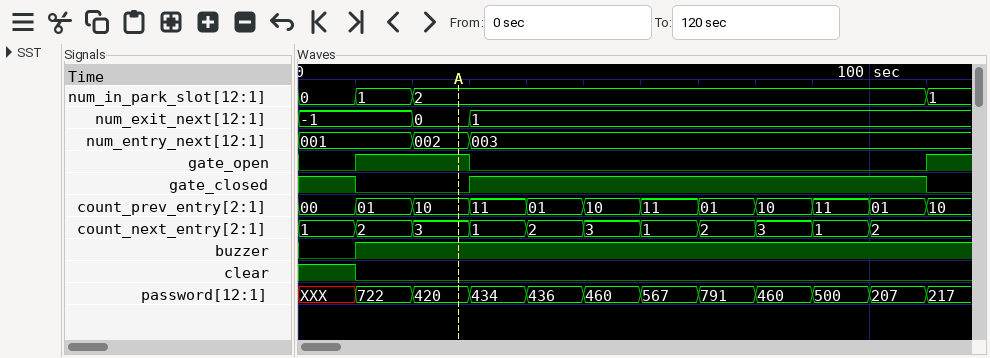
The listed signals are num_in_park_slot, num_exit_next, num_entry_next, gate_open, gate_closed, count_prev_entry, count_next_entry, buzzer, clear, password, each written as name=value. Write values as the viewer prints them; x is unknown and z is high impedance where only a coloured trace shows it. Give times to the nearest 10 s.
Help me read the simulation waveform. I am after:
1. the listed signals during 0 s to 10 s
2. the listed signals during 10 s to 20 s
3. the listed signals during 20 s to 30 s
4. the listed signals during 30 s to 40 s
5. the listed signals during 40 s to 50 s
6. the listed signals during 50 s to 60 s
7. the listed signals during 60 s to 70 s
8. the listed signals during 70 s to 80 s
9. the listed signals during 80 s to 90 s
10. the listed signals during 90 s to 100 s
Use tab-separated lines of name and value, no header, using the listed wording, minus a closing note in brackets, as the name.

the listed signals during 0 s to 10 s	num_in_park_slot=0, num_exit_next=-1, num_entry_next=001, gate_open=0, gate_closed=1, count_prev_entry=00, count_next_entry=1, buzzer=0, clear=1, password=XXX
the listed signals during 10 s to 20 s	num_in_park_slot=1, num_exit_next=-1, num_entry_next=001, gate_open=1, gate_closed=0, count_prev_entry=01, count_next_entry=2, buzzer=1, clear=0, password=722
the listed signals during 20 s to 30 s	num_in_park_slot=2, num_exit_next=0, num_entry_next=002, gate_open=1, gate_closed=0, count_prev_entry=10, count_next_entry=3, buzzer=1, clear=0, password=420
the listed signals during 30 s to 40 s	num_in_park_slot=2, num_exit_next=1, num_entry_next=003, gate_open=0, gate_closed=1, count_prev_entry=11, count_next_entry=1, buzzer=1, clear=0, password=434
the listed signals during 40 s to 50 s	num_in_park_slot=2, num_exit_next=1, num_entry_next=003, gate_open=0, gate_closed=1, count_prev_entry=01, count_next_entry=2, buzzer=1, clear=0, password=436
the listed signals during 50 s to 60 s	num_in_park_slot=2, num_exit_next=1, num_entry_next=003, gate_open=0, gate_closed=1, count_prev_entry=10, count_next_entry=3, buzzer=1, clear=0, password=460
the listed signals during 60 s to 70 s	num_in_park_slot=2, num_exit_next=1, num_entry_next=003, gate_open=0, gate_closed=1, count_prev_entry=11, count_next_entry=1, buzzer=1, clear=0, password=567
the listed signals during 70 s to 80 s	num_in_park_slot=2, num_exit_next=1, num_entry_next=003, gate_open=0, gate_closed=1, count_prev_entry=01, count_next_entry=2, buzzer=1, clear=0, password=791
the listed signals during 80 s to 90 s	num_in_park_slot=2, num_exit_next=1, num_entry_next=003, gate_open=0, gate_closed=1, count_prev_entry=10, count_next_entry=3, buzzer=1, clear=0, password=460
the listed signals during 90 s to 100 s	num_in_park_slot=2, num_exit_next=1, num_entry_next=003, gate_open=0, gate_closed=1, count_prev_entry=11, count_next_entry=1, buzzer=1, clear=0, password=500
